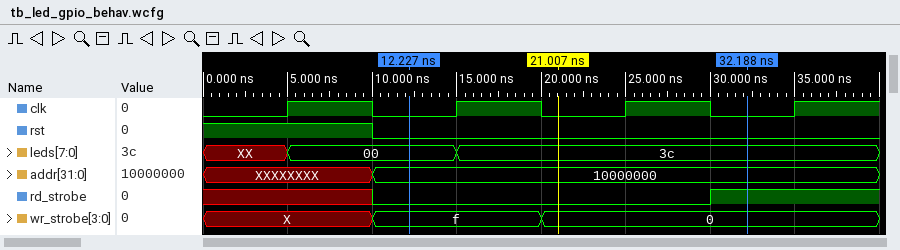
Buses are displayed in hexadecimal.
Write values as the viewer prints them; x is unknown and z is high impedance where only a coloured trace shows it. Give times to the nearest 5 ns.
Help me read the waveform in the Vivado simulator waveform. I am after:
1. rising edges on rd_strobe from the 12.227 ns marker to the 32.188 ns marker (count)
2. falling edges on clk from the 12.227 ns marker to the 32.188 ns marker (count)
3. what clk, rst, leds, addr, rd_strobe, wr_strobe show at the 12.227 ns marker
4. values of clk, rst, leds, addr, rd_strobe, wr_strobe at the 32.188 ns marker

1
2
clk=0, rst=0, leds=00, addr=10000000, rd_strobe=0, wr_strobe=f
clk=0, rst=0, leds=3c, addr=10000000, rd_strobe=1, wr_strobe=0
